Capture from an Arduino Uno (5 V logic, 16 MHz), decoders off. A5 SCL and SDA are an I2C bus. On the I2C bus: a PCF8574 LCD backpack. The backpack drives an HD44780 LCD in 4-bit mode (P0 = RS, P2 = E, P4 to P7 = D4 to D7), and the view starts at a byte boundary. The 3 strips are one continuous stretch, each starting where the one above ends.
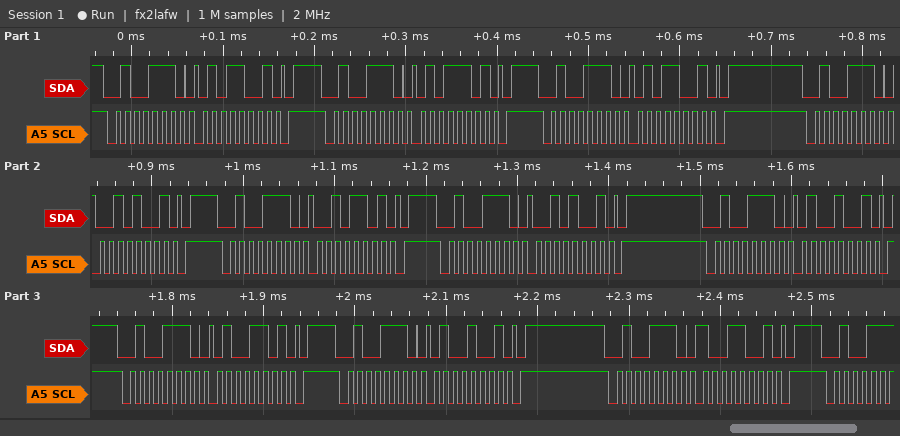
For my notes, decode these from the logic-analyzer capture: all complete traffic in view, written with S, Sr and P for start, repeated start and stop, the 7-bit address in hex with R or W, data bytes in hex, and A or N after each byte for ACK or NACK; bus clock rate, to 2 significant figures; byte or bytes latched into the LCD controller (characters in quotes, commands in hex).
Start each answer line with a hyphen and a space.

- S 27W A 59 A P S 27W A 5D A P S 27W A 59 A P S 27W A 29 A P S 27W A 2D A P S 27W A 29 A P S 27W A 49 A P S 27W A 4D A P S 27W A 49 A P S 27W A 99 A P
- 100 kHz
- 'R'
